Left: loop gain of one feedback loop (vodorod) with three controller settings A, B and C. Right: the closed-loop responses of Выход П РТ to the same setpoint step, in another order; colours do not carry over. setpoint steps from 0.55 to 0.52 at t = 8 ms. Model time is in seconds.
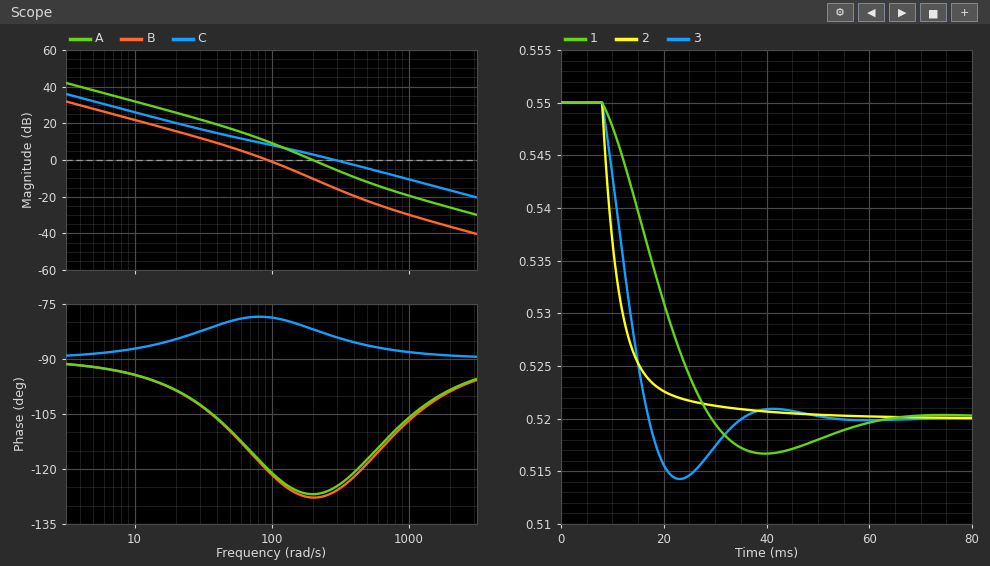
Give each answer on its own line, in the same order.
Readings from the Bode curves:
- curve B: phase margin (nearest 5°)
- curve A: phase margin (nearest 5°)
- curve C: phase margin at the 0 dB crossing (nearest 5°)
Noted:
60°
55°
95°
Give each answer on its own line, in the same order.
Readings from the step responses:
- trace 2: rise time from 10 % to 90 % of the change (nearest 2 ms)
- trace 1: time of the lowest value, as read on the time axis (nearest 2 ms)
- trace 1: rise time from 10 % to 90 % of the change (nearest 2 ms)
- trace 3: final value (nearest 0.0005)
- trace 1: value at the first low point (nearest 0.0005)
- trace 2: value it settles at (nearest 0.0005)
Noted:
10 ms
40 ms
16 ms
0.5200
0.5165
0.5200
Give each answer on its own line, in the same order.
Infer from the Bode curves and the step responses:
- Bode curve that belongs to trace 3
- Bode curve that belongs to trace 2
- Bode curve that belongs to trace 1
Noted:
A
C
B
